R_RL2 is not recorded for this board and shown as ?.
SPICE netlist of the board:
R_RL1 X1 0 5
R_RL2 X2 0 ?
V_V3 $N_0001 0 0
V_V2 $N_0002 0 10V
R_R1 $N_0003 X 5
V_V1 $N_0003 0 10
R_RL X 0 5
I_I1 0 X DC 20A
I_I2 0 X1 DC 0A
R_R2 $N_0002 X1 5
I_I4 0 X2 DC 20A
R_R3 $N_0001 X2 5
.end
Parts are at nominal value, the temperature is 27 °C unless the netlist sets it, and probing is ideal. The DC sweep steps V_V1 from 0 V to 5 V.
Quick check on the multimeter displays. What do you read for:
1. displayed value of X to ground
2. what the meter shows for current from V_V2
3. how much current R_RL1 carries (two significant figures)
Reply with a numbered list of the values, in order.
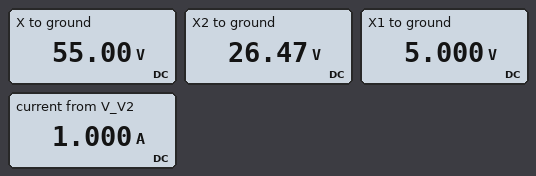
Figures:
1. 55.00 V
2. 1.000 A
3. 1.0 A
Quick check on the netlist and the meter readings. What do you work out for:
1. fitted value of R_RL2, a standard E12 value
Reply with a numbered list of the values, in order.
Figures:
1. 1.8 Ω
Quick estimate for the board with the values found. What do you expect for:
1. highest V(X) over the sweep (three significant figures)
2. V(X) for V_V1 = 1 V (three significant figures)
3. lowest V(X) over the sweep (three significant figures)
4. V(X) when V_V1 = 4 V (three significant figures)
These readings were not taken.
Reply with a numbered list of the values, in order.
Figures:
1. 52.5 V
2. 50.5 V
3. 50.0 V
4. 52.0 V
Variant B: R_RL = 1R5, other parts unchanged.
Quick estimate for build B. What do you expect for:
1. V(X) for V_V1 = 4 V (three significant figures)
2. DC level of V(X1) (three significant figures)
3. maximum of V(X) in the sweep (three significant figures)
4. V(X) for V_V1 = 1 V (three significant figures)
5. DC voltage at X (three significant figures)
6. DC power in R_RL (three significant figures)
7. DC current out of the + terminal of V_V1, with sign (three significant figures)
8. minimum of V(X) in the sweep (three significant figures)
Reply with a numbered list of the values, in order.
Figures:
1. 24.0 V
2. 5.00 V
3. 24.2 V
4. 23.3 V
5. 25.4 V
6. 430 W
7. -3.08 A
8. 23.1 V
